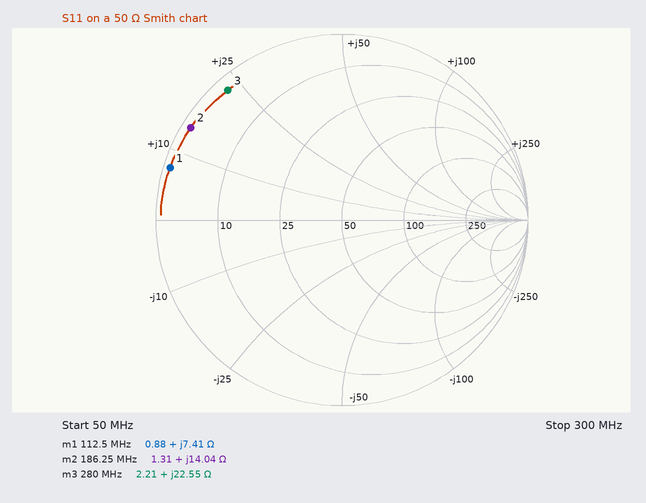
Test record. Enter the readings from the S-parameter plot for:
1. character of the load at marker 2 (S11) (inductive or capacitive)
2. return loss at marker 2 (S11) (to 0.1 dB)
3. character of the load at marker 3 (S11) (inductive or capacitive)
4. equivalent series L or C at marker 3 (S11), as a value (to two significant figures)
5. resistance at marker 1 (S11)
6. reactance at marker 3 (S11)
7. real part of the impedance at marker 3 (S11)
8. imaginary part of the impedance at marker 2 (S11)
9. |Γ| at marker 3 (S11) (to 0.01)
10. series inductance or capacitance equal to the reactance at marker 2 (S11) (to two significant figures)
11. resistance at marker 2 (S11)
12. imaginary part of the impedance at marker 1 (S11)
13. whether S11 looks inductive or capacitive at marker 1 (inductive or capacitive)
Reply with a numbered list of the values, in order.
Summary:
1. inductive
2. 0.4 dB
3. inductive
4. 13 nH
5. 0.88 Ω
6. +22.55 Ω
7. 2.21 Ω
8. +14.04 Ω
9. 0.93
10. 12 nH
11. 1.31 Ω
12. +7.41 Ω
13. inductive
